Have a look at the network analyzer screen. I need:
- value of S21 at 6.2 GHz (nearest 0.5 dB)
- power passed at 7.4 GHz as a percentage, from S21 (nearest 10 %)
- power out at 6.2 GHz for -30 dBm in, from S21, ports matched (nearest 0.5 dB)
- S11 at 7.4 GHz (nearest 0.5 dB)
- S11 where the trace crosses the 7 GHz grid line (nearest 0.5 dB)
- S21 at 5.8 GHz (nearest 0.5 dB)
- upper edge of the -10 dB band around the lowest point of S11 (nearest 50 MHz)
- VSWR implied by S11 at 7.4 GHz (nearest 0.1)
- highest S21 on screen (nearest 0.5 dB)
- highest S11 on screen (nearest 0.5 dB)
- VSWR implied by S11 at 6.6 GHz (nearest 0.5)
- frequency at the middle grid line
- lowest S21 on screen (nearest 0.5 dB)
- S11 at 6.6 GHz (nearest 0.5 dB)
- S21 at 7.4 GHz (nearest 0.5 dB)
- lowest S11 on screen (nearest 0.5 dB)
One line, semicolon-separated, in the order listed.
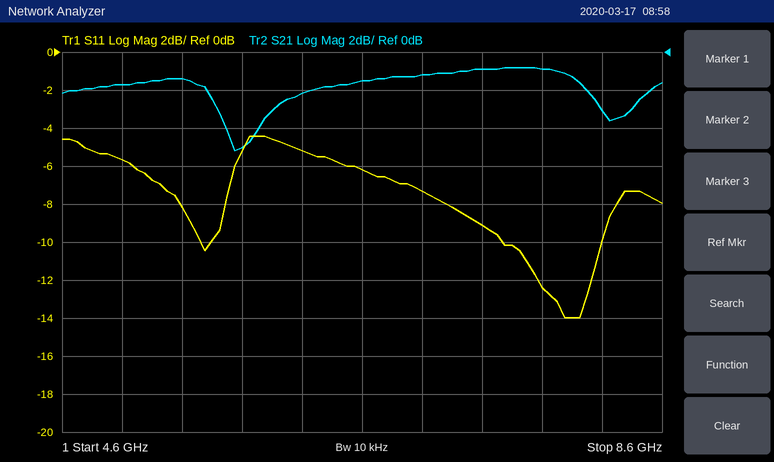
-2.0 dB; 80 %; -32.0 dBm; -9.0 dB; -7.5 dB; -5.0 dB; 8.20 GHz; 2.1; -1.0 dB; -4.5 dB; 3.0; 6.6 GHz; -5.0 dB; -6.0 dB; -1.0 dB; -14.0 dB
